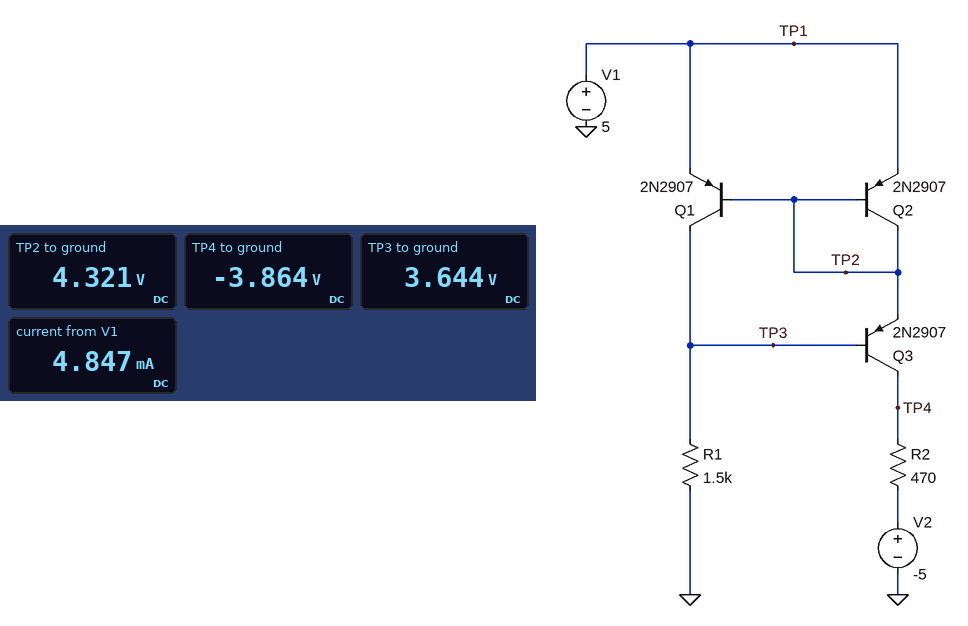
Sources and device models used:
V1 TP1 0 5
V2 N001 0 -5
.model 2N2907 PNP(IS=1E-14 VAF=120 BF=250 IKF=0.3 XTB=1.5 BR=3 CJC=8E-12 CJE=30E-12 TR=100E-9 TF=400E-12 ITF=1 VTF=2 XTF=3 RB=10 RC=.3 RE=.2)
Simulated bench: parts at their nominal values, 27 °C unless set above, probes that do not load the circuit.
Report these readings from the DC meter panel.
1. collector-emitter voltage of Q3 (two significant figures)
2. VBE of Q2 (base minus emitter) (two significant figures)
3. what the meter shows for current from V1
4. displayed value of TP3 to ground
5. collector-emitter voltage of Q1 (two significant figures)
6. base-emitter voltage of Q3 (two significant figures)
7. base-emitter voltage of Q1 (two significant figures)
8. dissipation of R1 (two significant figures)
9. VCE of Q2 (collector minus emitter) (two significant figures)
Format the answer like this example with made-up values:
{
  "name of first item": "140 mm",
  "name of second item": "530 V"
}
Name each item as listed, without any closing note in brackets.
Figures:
{
  "collector-emitter voltage of Q3": "-8.2 V",
  "VBE of Q2 (base minus emitter)": "-680 mV",
  "what the meter shows for current from V1": "4.847 mA",
  "displayed value of TP3 to ground": "3.644 V",
  "collector-emitter voltage of Q1": "-1.4 V",
  "base-emitter voltage of Q3": "-680 mV",
  "base-emitter voltage of Q1": "-680 mV",
  "dissipation of R1": "8.9 mW",
  "VCE of Q2 (collector minus emitter)": "-680 mV"
}
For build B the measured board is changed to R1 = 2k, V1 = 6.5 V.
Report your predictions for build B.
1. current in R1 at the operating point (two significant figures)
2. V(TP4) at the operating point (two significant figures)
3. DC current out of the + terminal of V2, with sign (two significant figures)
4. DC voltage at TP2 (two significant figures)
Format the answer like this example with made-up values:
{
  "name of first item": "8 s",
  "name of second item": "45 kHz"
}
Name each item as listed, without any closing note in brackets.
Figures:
{
  "current in R1 at the operating point": "2.6 mA",
  "V(TP4) at the operating point": "-3.8 V",
  "DC current out of the + terminal of V2, with sign": "-2.6 mA",
  "DC voltage at TP2": "5.8 V"
}
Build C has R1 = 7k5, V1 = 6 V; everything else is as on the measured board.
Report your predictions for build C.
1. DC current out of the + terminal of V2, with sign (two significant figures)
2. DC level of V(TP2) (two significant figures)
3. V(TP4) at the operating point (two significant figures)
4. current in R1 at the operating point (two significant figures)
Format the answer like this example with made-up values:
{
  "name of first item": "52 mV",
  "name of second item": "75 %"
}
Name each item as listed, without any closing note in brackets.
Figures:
{
  "DC current out of the + terminal of V2, with sign": "-630 µA",
  "DC level of V(TP2)": "5.4 V",
  "V(TP4) at the operating point": "-4.7 V",
  "current in R1 at the operating point": "630 µA"
}
